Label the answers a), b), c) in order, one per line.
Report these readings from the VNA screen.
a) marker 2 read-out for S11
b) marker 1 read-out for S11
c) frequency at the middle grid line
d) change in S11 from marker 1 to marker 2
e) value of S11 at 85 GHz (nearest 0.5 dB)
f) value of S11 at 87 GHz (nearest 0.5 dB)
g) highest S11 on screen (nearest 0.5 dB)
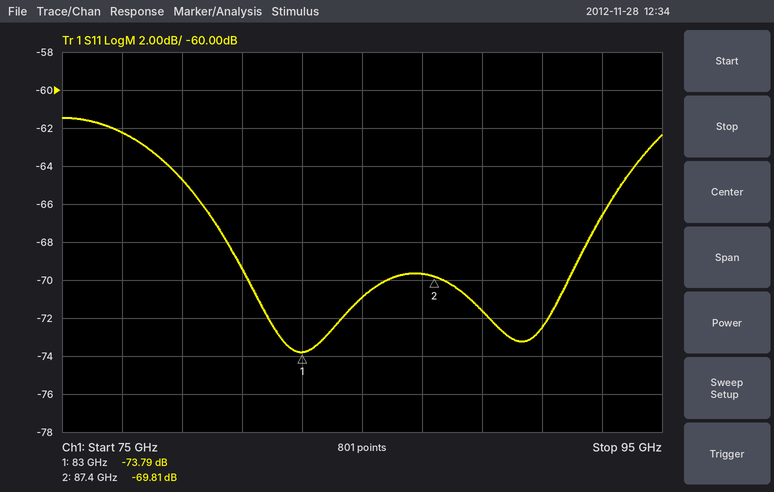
a) -69.81 dB
b) -73.79 dB
c) 85 GHz
d) 3.98 dB
e) -71.0 dB
f) -69.5 dB
g) -61.5 dB
